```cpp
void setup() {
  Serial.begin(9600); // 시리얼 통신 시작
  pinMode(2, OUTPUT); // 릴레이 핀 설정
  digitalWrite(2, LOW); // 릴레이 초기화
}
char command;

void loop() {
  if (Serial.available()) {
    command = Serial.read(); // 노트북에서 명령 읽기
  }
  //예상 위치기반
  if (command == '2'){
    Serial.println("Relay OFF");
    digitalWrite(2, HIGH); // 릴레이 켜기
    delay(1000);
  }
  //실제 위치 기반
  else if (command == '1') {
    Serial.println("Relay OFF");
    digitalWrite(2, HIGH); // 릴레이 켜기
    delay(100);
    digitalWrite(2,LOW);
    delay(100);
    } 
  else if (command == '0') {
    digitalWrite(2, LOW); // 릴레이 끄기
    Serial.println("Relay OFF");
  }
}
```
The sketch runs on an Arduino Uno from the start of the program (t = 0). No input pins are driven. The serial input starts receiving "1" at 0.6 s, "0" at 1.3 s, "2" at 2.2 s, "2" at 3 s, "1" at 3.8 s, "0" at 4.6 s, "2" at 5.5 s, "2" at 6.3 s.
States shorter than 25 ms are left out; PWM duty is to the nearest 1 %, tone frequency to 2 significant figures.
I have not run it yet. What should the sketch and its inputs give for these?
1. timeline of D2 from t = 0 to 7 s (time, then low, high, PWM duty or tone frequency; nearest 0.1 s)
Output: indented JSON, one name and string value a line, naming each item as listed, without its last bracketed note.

{
  "timeline of D2 from t = 0 to 7 s": "0 s low; 0.6 s high; 0.7 s low; 0.8 s high; 0.9 s low; 1 s high; 1.1 s low; 1.2 s high; 1.3 s low; 2.2 s high; 4.3 s low; 4.4 s high; 4.5 s low; 5.5 s high"
}
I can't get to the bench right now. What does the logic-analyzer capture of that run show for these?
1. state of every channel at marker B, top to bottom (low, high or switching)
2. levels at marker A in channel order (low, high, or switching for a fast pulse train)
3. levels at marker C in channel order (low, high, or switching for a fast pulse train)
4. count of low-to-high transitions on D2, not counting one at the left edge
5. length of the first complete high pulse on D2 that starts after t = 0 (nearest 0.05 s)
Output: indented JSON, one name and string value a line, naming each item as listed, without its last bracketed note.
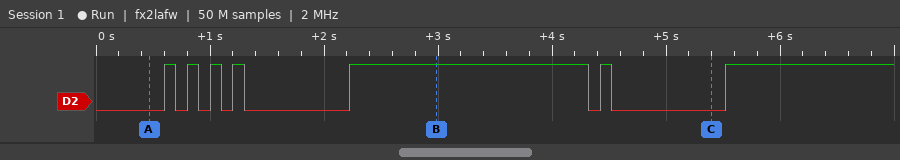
{
  "state of every channel at marker B, top to bottom": "D2 high",
  "levels at marker A in channel order": "D2 low",
  "levels at marker C in channel order": "D2 low",
  "count of low-to-high transitions on D2, not counting one at the left edge": "7",
  "length of the first complete high pulse on D2 that starts after t = 0": "0.10 s"
}
